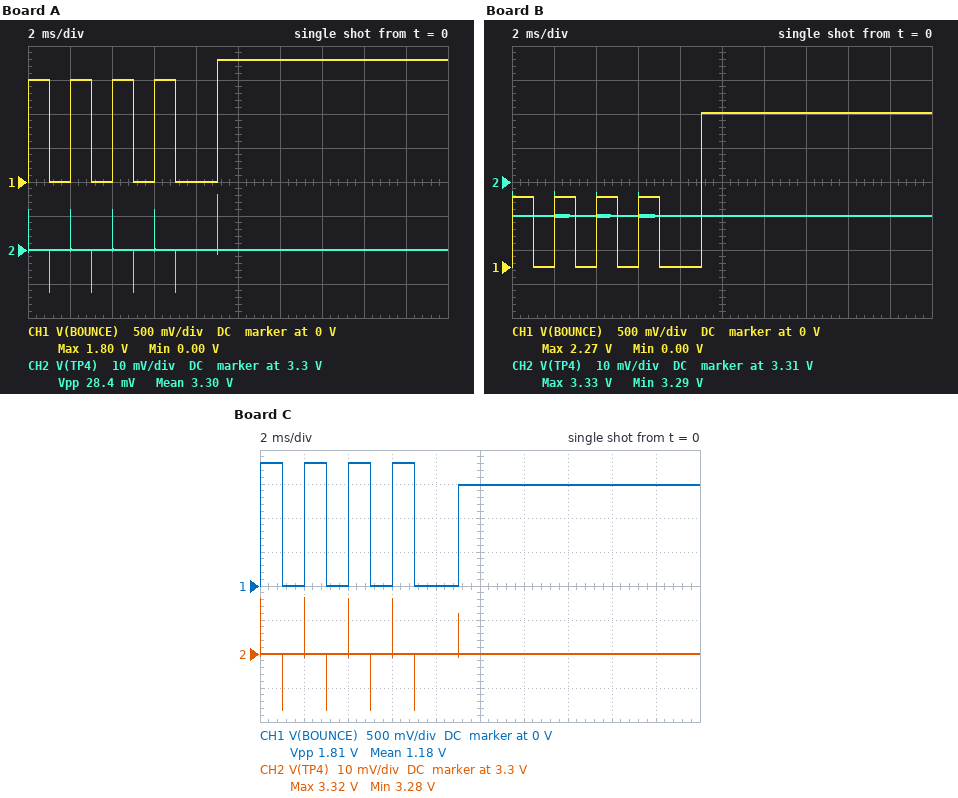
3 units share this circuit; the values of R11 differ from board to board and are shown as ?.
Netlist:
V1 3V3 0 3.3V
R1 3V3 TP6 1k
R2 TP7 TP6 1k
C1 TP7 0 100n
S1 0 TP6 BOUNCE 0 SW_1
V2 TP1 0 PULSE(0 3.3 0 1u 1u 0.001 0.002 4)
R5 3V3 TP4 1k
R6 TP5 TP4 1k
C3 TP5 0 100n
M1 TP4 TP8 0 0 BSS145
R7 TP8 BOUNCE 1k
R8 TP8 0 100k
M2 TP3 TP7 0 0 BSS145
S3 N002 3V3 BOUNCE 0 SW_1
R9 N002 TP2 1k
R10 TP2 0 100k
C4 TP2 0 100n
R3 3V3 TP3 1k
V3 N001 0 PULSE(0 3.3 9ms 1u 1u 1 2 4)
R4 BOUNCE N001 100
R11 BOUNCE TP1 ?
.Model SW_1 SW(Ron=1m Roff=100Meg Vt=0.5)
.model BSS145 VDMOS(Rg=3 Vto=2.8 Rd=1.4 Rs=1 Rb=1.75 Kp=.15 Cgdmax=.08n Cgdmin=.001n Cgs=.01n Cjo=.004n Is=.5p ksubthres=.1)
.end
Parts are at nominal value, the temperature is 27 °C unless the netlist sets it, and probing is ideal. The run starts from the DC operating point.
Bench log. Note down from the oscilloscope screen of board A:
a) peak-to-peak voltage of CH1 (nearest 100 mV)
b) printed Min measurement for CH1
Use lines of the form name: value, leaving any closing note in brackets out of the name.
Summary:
peak-to-peak voltage of CH1: 1.8 V
printed Min measurement for CH1: 0.00 V
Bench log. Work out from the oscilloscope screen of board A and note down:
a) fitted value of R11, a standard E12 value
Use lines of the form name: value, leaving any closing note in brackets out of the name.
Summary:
fitted value of R11, a standard E12 value: 120 Ω
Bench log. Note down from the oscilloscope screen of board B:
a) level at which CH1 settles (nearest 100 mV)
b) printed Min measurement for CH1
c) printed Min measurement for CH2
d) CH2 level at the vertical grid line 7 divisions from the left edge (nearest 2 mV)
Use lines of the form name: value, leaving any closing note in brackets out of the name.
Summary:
level at which CH1 settles: 2.3 V
printed Min measurement for CH1: 0.00 V
printed Min measurement for CH2: 3.29 V
CH2 level at the vertical grid line 7 divisions from the left edge: 3.300 V
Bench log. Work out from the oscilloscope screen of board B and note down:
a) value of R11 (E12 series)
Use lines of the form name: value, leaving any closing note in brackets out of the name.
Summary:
value of R11: 220 Ω
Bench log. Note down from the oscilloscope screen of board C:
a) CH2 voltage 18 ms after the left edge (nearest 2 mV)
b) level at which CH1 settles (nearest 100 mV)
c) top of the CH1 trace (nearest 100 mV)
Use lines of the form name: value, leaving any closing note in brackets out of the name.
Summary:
CH2 voltage 18 ms after the left edge: 3.300 V
level at which CH1 settles: 1.5 V
top of the CH1 trace: 1.8 V
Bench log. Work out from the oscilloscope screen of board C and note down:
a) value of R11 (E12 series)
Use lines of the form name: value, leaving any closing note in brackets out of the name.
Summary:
value of R11: 82 Ω
